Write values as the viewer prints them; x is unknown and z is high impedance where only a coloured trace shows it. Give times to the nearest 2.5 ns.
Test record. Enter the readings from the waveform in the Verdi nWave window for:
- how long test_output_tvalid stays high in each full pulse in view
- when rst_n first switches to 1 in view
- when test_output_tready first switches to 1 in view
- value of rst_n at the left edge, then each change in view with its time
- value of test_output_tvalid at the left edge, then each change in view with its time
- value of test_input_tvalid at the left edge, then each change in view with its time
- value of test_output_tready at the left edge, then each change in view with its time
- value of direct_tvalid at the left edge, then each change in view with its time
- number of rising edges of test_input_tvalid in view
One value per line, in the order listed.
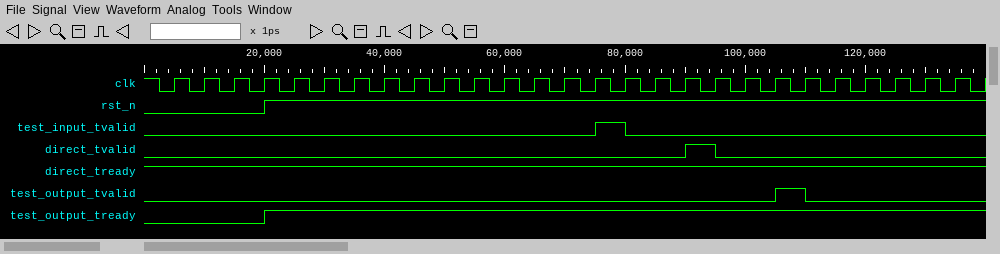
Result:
5 ns
20 ns
20 ns
0, 1 at 20 ns
0, 1 at 105 ns, 0 at 110 ns
0, 1 at 75 ns, 0 at 80 ns
0, 1 at 20 ns
0, 1 at 90 ns, 0 at 95 ns
1
